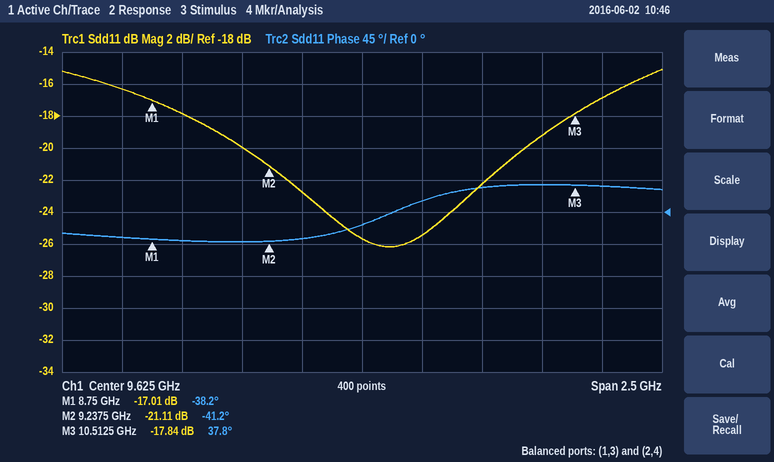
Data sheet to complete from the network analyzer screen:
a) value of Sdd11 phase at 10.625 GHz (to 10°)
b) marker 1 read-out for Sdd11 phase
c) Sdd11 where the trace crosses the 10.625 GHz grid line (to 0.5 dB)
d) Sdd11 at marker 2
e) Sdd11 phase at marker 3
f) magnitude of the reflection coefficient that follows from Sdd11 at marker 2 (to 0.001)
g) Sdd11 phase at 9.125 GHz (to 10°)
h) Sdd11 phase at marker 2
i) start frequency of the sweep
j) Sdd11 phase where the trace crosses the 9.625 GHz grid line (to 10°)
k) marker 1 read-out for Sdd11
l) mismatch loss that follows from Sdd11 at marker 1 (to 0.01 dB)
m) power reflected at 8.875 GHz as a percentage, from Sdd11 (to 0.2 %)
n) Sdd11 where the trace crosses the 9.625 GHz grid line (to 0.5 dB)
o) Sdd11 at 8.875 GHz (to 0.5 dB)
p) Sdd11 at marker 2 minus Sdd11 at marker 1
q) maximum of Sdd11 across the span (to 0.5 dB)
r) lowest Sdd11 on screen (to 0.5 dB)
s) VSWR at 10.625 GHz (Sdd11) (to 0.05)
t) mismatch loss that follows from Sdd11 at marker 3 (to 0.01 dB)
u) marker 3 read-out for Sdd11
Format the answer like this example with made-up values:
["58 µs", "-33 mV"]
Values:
["40°", "-38.2°", "-17.0 dB", "-21.11 dB", "37.8°", "0.088", "-40°", "-41.2°", "8.375 GHz", "-20°", "-17.01 dB", "0.09 dB", "1.6 %", "-25.5 dB", "-18.0 dB", "-4.10 dB", "-15.0 dB", "-26.0 dB", "1.35", "0.07 dB", "-17.84 dB"]
